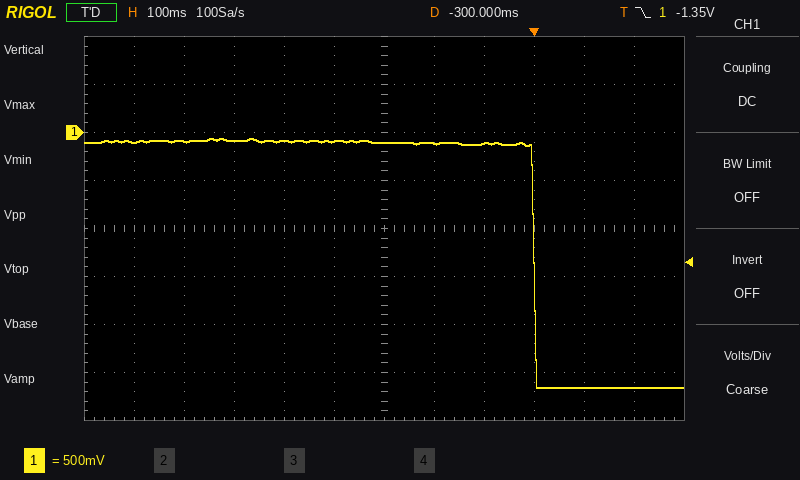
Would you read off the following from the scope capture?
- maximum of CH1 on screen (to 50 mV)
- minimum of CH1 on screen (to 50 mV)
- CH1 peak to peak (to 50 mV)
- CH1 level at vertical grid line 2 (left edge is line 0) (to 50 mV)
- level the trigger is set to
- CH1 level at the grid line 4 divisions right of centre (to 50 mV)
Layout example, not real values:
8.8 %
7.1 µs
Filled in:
-50 mV
-2.65 V
2.60 V
-100 mV
-1.35 V
-2.65 V
